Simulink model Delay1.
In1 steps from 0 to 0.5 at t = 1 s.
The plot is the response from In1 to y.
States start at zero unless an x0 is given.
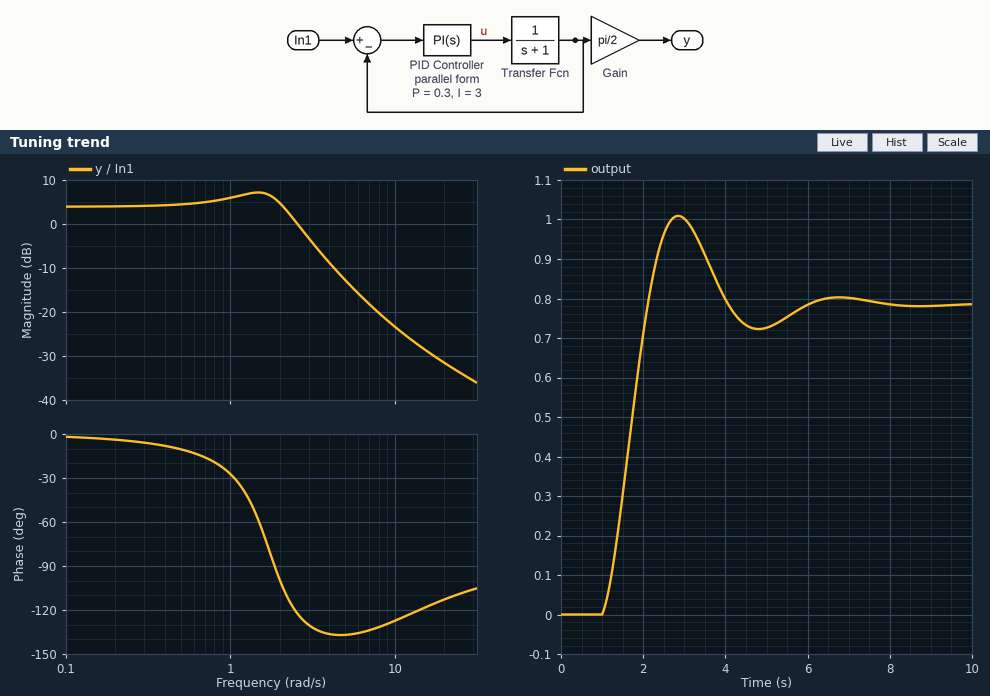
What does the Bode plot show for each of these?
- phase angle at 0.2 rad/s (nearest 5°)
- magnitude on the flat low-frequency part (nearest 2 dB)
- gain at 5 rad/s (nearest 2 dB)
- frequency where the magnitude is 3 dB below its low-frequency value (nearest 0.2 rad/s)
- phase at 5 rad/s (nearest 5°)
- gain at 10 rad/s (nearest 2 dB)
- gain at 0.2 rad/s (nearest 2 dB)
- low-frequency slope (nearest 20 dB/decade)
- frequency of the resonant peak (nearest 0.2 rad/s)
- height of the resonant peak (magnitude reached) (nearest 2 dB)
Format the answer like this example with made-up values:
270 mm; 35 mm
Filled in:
-5°; 4 dB; -12 dB; 2.4 rad/s; -135°; -24 dB; 4 dB; 0 dB/decade; 1.4 rad/s; 8 dB
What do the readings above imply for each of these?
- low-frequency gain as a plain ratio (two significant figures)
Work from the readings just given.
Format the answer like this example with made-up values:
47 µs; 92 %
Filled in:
1.6
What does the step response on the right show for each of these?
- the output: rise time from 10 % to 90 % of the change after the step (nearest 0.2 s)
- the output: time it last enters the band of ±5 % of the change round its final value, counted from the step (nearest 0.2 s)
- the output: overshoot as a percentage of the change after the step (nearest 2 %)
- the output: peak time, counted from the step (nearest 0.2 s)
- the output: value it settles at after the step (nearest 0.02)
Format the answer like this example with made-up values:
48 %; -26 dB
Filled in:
0.8 s; 4.4 s; 28 %; 1.8 s; 0.78
